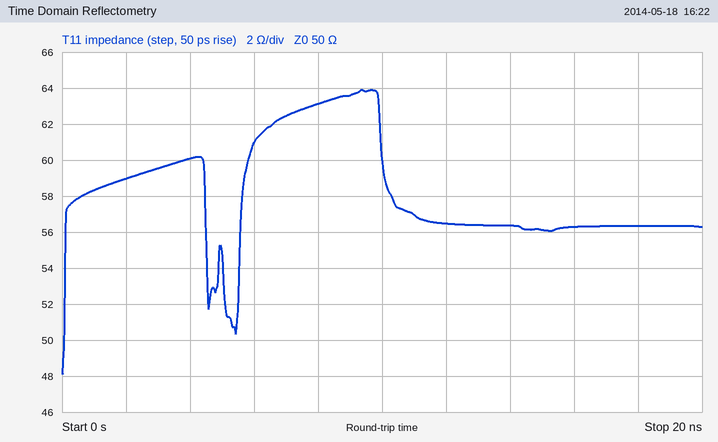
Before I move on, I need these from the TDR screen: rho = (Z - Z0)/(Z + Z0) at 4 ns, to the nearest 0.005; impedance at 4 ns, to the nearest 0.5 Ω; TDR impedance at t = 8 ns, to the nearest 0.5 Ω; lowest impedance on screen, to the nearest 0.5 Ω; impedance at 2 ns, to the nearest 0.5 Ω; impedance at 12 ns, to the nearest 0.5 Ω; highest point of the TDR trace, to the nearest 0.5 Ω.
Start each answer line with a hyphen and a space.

- +0.090
- 60.0 Ω
- 63.0 Ω
- 48.0 Ω
- 59.0 Ω
- 56.5 Ω
- 64.0 Ω
